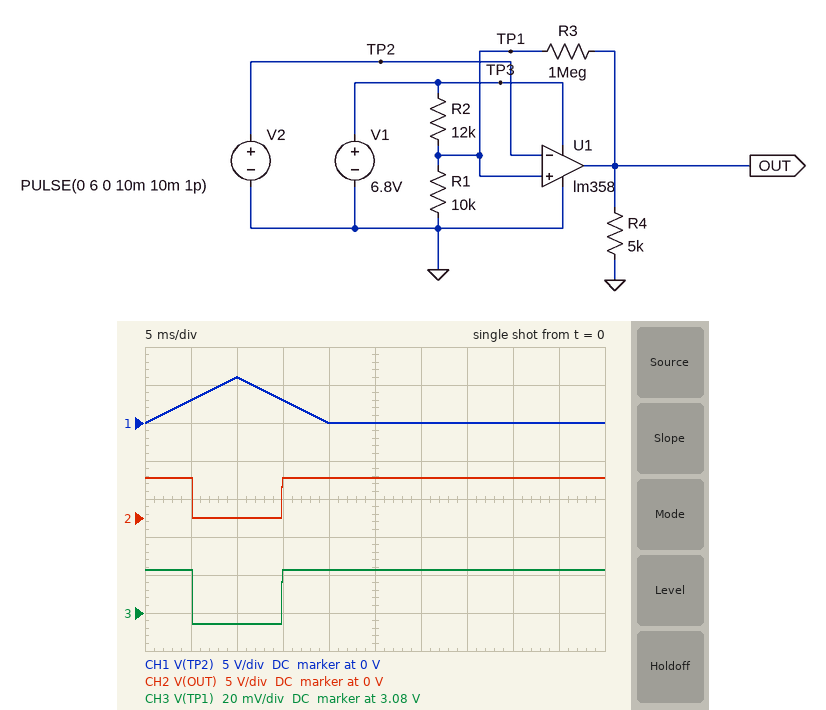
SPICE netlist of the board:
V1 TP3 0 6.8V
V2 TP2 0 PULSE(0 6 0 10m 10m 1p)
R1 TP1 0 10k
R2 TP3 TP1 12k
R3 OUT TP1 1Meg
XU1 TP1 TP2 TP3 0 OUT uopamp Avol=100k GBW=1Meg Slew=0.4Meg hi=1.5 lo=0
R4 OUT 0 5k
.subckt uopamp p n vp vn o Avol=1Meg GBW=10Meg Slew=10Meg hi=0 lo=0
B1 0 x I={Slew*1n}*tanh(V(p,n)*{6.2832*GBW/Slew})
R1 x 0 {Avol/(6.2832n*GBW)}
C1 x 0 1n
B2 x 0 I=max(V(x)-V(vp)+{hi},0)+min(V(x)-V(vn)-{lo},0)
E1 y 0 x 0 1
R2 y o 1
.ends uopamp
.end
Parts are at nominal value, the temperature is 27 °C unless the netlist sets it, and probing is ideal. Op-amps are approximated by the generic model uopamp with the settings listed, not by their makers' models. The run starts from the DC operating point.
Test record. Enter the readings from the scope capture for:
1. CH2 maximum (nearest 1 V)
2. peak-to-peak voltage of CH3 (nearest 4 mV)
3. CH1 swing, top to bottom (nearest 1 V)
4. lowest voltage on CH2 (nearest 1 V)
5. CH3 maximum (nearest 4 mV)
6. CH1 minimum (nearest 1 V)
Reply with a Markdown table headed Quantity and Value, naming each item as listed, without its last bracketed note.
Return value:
| Quantity | Value |
|---|---|
| CH2 maximum | 5 V |
| peak-to-peak voltage of CH3 | 28 mV |
| CH1 swing, top to bottom | 6 V |
| lowest voltage on CH2 | 0 V |
| CH3 maximum | 3.104 V |
| CH1 minimum | 0 V |
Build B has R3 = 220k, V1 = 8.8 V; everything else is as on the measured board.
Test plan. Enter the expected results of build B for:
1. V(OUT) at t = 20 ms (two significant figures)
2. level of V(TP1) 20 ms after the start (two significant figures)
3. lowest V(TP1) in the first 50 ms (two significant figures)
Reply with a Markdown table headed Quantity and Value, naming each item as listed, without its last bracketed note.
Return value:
| Quantity | Value |
|---|---|
| V(OUT) at t = 20 ms | 7.3 V |
| level of V(TP1) 20 ms after the start | 4.1 V |
| lowest V(TP1) in the first 50 ms | 3.9 V |
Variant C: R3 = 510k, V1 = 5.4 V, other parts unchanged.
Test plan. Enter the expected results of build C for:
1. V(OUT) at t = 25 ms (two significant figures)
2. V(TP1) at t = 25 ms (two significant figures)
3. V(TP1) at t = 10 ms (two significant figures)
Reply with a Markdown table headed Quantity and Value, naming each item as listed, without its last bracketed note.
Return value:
| Quantity | Value |
|---|---|
| V(OUT) at t = 25 ms | 3.9 V |
| V(TP1) at t = 25 ms | 2.5 V |
| V(TP1) at t = 10 ms | 2.4 V |
